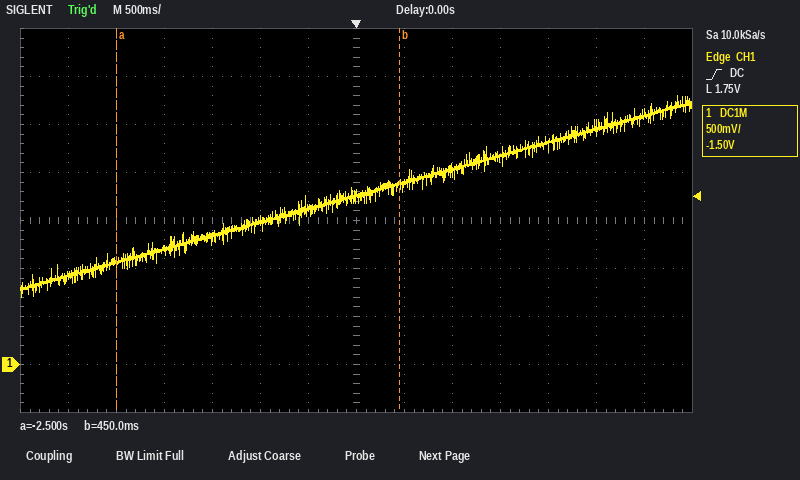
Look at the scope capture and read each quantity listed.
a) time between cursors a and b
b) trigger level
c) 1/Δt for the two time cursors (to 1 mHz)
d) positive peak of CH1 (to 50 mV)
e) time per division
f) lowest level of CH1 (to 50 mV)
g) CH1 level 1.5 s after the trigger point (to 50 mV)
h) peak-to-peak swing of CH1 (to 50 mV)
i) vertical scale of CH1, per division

2.95 s
1.75 V
339 mHz
2.80 V
500 ms
700 mV
2.15 V
2.10 V
500 mV
